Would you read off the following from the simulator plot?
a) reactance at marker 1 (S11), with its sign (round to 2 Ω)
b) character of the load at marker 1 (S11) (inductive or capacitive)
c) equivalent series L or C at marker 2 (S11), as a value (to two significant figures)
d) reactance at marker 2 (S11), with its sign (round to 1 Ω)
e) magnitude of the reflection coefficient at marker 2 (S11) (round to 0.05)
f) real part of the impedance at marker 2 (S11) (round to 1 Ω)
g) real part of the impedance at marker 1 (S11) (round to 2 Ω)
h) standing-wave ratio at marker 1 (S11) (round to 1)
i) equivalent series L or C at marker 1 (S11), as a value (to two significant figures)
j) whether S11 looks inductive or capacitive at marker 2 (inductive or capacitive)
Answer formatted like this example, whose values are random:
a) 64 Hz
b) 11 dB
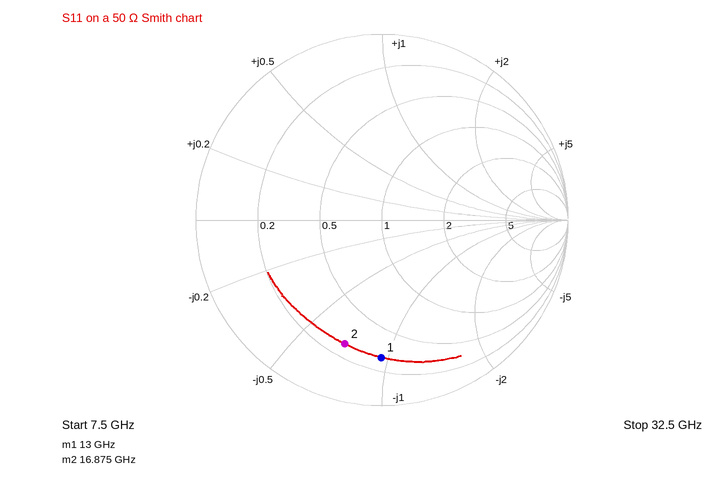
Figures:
a) -48 Ω
b) capacitive
c) 270 fF
d) -35 Ω
e) 0.70
f) 14 Ω
g) 14 Ω
h) 7
i) 260 fF
j) capacitive
